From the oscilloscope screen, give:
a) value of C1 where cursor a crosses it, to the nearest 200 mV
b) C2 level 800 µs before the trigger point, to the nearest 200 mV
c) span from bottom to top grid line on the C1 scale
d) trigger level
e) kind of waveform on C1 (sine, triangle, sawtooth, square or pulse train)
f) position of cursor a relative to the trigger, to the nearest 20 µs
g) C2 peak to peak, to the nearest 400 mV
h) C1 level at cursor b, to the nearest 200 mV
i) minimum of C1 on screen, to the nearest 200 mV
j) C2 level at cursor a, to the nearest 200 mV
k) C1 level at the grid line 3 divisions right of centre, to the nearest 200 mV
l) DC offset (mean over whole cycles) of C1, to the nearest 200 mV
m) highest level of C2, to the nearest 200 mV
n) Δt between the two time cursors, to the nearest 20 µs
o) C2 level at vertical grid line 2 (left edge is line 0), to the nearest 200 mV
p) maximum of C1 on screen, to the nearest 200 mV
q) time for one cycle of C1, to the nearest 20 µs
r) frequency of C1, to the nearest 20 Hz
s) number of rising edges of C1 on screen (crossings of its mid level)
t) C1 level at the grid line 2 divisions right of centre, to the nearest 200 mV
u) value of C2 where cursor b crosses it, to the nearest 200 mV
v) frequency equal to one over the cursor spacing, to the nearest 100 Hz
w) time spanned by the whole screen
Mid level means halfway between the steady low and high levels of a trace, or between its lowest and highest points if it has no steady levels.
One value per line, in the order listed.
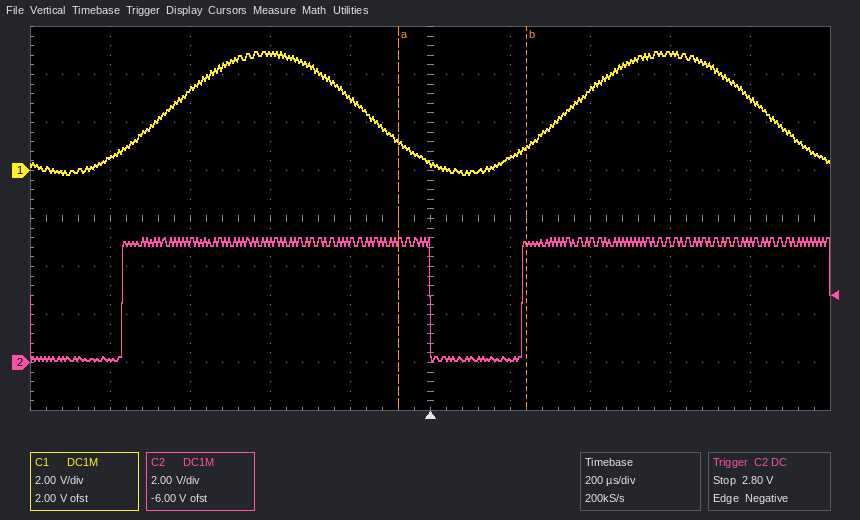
1.2 V
200 mV
16 V
2.80 V
sine
-80 µs
5.2 V
1.0 V
-200 mV
5.0 V
4.8 V
2.4 V
5.2 V
320 µs
5.0 V
5.0 V
1.00 ms
1.00 kHz
2
3.4 V
5.0 V
3.1 kHz
2 ms
